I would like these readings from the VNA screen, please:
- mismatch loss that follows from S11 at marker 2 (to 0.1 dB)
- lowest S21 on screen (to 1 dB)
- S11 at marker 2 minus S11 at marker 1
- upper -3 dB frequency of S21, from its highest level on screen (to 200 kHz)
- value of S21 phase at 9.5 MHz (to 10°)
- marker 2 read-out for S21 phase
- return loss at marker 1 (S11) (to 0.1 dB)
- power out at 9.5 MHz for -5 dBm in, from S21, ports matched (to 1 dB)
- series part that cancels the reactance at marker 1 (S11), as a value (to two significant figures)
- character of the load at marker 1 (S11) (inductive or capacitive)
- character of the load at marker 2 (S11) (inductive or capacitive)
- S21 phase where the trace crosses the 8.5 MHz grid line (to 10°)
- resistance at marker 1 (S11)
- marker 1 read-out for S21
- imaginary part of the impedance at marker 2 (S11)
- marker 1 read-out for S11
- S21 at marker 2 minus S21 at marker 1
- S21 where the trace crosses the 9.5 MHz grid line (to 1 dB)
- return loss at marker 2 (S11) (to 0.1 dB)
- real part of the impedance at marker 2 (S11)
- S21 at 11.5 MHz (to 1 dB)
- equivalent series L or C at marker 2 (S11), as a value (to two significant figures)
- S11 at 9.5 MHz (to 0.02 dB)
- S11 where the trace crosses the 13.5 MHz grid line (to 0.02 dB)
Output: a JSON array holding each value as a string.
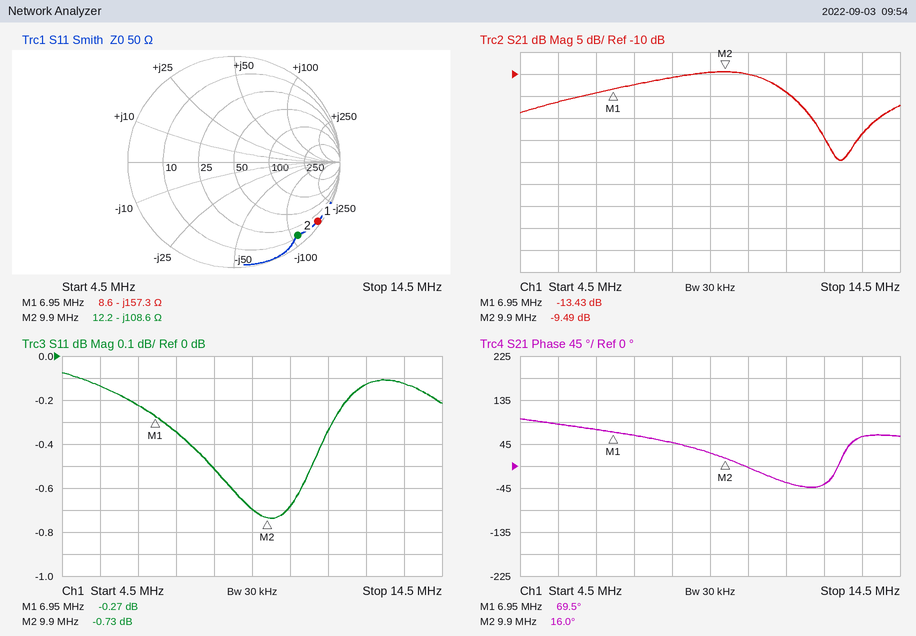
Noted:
["8.1 dB", "-30 dB", "-0.46 dB", "11.2 MHz", "30°", "16.0°", "0.3 dB", "-15 dBm", "3.6 µH", "capacitive", "capacitive", "50°", "8.6 Ω", "-13.43 dB", "-108.6 Ω", "-0.27 dB", "3.94 dB", "-10 dB", "0.7 dB", "12.2 Ω", "-14 dB", "150 pF", "-0.70 dB", "-0.12 dB"]
